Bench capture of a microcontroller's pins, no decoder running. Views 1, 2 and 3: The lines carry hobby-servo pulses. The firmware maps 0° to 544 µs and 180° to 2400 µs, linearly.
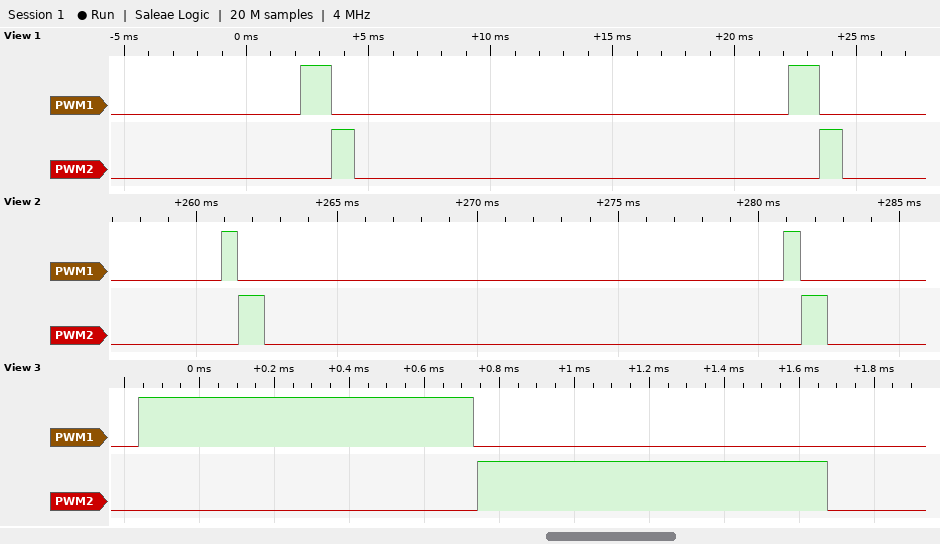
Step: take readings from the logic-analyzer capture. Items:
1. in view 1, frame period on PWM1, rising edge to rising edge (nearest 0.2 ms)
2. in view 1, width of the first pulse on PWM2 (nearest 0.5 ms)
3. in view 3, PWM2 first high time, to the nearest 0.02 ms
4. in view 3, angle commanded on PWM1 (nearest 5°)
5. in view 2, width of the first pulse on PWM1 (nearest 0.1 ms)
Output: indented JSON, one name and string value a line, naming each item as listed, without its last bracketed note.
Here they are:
{
  "in view 1, frame period on PWM1, rising edge to rising edge": "20.0 ms",
  "in view 1, width of the first pulse on PWM2": "1.0 ms",
  "in view 3, PWM2 first high time, to the nearest 0.02 ms": "0.94 ms",
  "in view 3, angle commanded on PWM1": "35°",
  "in view 2, width of the first pulse on PWM1": "0.6 ms"
}
